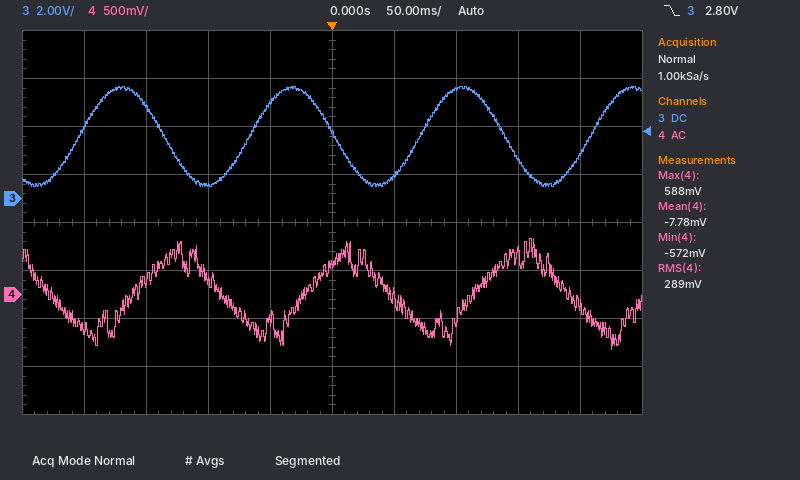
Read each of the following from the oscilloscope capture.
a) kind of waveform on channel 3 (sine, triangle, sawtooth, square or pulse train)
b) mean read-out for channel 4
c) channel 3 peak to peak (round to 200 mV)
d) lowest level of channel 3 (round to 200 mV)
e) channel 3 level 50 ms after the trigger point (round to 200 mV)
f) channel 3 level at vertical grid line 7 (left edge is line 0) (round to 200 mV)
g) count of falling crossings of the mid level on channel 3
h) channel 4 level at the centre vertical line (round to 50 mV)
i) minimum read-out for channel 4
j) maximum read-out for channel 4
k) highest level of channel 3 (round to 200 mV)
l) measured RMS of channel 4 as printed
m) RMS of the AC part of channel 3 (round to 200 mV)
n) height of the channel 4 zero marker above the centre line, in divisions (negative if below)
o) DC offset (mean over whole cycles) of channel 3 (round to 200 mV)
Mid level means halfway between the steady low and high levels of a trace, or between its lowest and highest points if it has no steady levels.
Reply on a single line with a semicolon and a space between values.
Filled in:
sine; -7.78 mV; 4.2 V; 400 mV; 1.0 V; 4.6 V; 3; 300 mV; -572 mV; 588 mV; 4.6 V; 289 mV; 1.4 V; -1.5 div; 2.6 V
